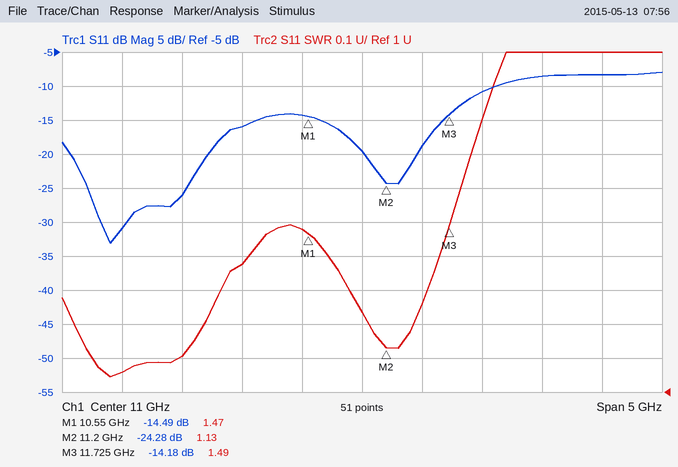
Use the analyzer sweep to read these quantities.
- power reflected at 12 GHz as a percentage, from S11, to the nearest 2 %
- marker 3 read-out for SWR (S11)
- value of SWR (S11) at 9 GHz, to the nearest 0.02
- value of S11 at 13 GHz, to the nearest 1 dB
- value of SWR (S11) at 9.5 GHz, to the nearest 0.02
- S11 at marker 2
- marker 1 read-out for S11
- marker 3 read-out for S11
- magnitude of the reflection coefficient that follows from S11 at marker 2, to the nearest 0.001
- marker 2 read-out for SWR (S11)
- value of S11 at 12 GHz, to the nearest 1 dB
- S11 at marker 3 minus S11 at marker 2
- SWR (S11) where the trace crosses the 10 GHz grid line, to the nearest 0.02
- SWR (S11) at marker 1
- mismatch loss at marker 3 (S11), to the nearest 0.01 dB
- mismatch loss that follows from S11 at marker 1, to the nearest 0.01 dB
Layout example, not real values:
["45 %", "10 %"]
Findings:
["8 %", "1.49", "1.06", "-8 dB", "1.10", "-24.28 dB", "-14.49 dB", "-14.18 dB", "0.061", "1.13", "-11 dB", "10.10 dB", "1.38", "1.47", "0.17 dB", "0.16 dB"]
